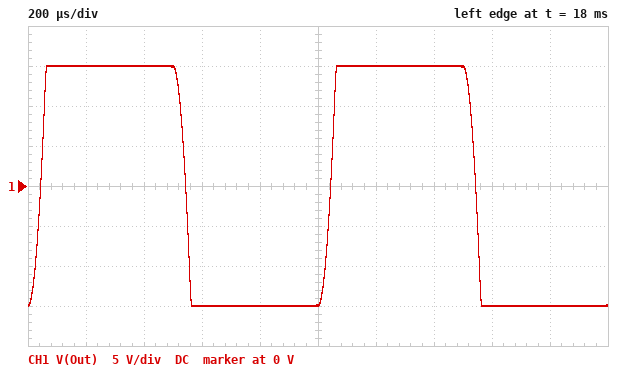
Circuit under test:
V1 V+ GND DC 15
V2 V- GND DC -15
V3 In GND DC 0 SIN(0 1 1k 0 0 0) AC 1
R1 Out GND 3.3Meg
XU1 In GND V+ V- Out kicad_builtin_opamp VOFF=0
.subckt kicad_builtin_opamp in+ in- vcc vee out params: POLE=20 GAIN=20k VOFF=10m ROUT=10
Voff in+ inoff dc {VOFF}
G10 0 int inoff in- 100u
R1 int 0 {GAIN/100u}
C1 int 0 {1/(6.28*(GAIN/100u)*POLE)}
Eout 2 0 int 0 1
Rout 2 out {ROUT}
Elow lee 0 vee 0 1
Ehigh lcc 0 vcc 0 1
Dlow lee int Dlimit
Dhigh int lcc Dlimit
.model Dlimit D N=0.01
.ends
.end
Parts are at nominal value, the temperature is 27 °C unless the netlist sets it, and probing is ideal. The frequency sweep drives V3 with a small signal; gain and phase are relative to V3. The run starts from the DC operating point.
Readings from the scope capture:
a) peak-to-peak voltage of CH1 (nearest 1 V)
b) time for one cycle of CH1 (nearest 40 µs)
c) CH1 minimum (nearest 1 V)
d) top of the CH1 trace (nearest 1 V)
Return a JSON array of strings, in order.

["30 V", "1.00 ms", "-15 V", "15 V"]
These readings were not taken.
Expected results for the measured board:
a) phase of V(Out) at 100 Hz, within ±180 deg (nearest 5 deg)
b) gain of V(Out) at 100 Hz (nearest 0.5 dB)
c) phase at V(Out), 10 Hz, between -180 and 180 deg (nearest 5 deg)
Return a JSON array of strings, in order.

["-80 deg", "72.0 dB", "-25 deg"]
